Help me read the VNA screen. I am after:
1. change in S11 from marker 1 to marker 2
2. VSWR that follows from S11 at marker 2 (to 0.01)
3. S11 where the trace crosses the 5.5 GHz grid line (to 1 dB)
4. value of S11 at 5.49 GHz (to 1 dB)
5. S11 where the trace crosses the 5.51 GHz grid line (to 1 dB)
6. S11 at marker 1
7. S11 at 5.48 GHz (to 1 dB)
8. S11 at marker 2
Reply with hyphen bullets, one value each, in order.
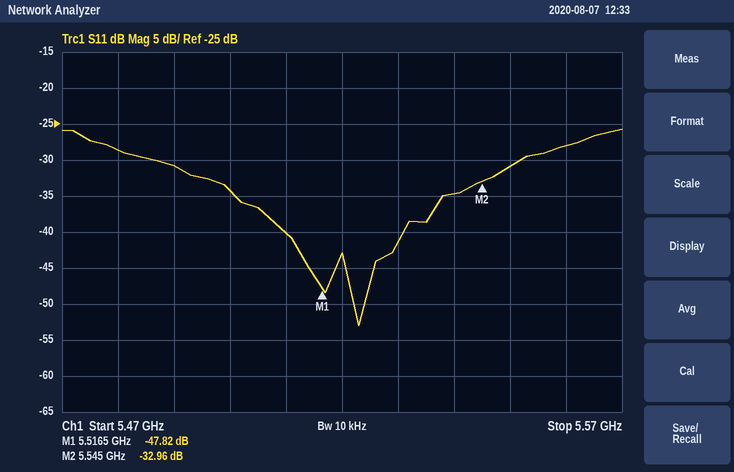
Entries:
- 14.86 dB
- 1.05
- -34 dB
- -31 dB
- -40 dB
- -47.82 dB
- -29 dB
- -32.96 dB
